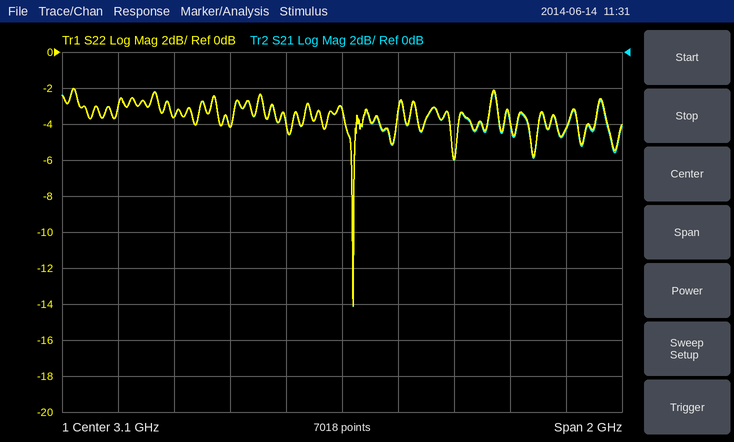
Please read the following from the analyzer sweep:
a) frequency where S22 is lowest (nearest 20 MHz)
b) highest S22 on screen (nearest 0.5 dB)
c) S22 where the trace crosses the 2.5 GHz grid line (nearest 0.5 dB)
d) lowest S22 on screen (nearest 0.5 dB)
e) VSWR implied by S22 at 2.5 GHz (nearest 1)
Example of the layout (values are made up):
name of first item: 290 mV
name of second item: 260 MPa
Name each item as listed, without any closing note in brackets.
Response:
frequency where S22 is lowest: 3.14 GHz
highest S22 on screen: -2.0 dB
S22 where the trace crosses the 2.5 GHz grid line: -3.5 dB
lowest S22 on screen: -14.0 dB
VSWR implied by S22 at 2.5 GHz: 5
